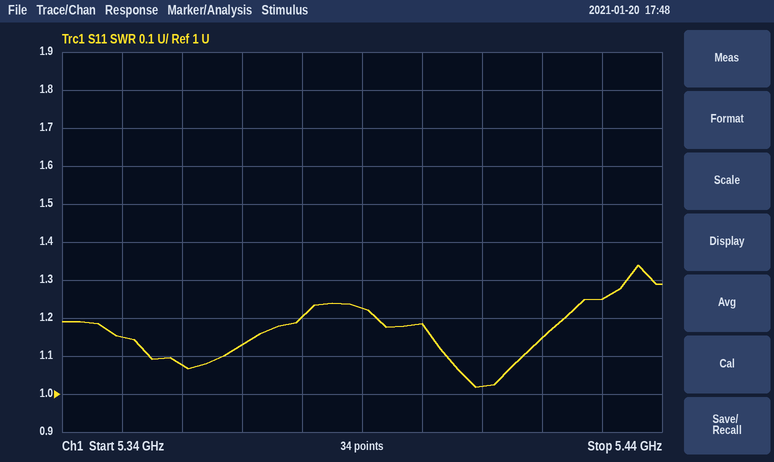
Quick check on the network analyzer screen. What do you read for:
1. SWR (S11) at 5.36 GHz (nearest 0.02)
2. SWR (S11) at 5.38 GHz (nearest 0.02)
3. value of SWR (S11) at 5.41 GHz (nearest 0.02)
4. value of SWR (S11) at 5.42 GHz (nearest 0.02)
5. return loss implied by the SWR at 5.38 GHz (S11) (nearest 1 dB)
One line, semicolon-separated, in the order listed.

1.08; 1.20; 1.02; 1.14; 21 dB
